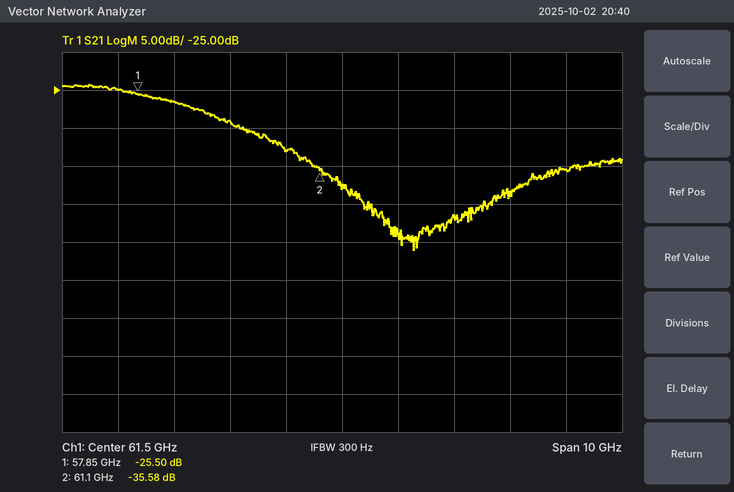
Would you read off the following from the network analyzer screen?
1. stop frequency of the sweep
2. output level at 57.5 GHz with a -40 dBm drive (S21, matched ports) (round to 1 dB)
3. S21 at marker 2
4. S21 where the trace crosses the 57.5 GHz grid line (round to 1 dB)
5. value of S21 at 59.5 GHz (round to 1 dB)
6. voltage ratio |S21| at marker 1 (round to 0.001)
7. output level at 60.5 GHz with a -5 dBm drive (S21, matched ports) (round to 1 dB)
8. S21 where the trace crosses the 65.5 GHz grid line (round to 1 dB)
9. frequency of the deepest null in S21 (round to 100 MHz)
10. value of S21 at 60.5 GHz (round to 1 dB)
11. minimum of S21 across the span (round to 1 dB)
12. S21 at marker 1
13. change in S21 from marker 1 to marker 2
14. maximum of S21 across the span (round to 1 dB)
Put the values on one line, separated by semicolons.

66.5 GHz; -65 dBm; -35.58 dB; -25 dB; -29 dB; 0.053; -38 dBm; -35 dB; 62.8 GHz; -33 dB; -46 dB; -25.50 dB; -10.08 dB; -24 dB
